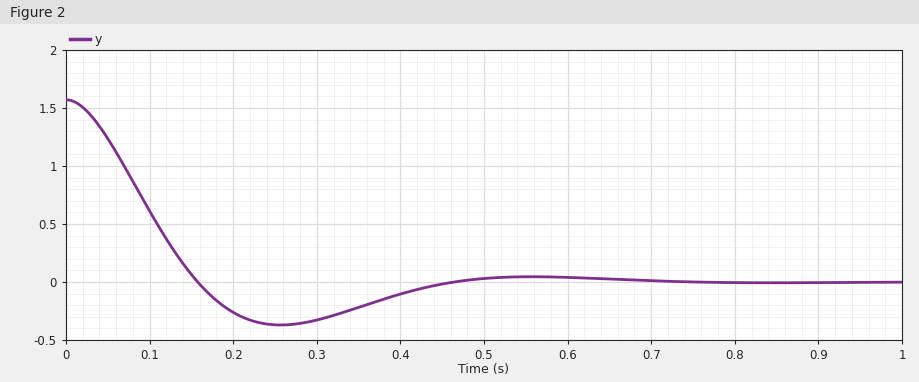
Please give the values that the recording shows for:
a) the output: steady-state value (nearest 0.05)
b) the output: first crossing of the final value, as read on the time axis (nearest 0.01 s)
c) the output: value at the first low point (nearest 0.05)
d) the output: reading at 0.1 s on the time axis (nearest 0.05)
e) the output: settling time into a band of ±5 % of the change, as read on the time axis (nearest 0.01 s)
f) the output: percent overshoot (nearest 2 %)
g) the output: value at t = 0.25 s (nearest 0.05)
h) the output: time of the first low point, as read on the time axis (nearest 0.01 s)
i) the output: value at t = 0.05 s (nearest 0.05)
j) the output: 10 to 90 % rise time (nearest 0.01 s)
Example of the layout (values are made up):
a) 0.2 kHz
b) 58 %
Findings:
a) 0.00
b) 0.16 s
c) -0.35
d) 0.60
e) 0.41 s
f) 24 %
g) -0.35
h) 0.26 s
i) 1.25
j) 0.11 s
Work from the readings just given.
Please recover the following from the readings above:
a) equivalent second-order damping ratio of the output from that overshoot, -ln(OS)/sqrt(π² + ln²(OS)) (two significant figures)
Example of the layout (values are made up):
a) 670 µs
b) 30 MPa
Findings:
a) 0.41
